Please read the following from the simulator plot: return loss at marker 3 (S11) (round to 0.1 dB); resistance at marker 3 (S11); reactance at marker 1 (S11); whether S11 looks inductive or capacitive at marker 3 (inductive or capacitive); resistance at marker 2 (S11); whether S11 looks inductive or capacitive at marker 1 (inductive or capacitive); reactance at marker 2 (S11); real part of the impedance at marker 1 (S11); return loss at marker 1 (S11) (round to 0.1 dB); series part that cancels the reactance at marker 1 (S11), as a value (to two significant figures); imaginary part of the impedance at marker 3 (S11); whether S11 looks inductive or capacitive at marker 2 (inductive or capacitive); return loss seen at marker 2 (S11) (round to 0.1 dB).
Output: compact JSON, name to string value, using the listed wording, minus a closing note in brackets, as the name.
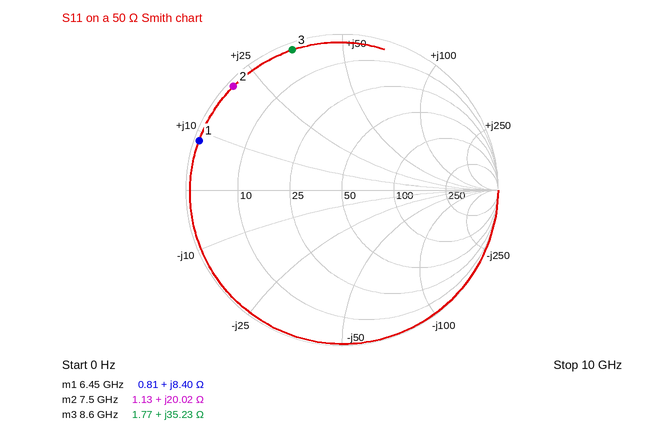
{"return loss at marker 3 (S11)": "0.4 dB", "resistance at marker 3": "1.77 Ω", "reactance at marker 1": "+8.40 Ω", "whether S11 looks inductive or capacitive at marker 3": "inductive", "resistance at marker 2": "1.13 Ω", "whether S11 looks inductive or capacitive at marker 1": "inductive", "reactance at marker 2": "+20.02 Ω", "real part of the impedance at marker 1": "0.81 Ω", "return loss at marker 1 (S11)": "0.3 dB", "series part that cancels the reactance at marker 1 (S11), as a value": "2.9 pF", "imaginary part of the impedance at marker 3": "+35.23 Ω", "whether S11 looks inductive or capacitive at marker 2": "inductive", "return loss seen at marker 2 (S11)": "0.3 dB"}
